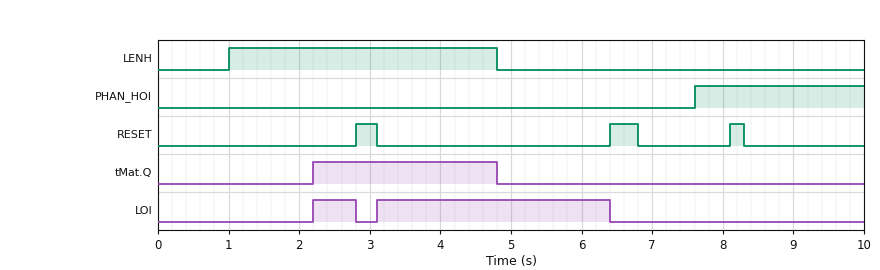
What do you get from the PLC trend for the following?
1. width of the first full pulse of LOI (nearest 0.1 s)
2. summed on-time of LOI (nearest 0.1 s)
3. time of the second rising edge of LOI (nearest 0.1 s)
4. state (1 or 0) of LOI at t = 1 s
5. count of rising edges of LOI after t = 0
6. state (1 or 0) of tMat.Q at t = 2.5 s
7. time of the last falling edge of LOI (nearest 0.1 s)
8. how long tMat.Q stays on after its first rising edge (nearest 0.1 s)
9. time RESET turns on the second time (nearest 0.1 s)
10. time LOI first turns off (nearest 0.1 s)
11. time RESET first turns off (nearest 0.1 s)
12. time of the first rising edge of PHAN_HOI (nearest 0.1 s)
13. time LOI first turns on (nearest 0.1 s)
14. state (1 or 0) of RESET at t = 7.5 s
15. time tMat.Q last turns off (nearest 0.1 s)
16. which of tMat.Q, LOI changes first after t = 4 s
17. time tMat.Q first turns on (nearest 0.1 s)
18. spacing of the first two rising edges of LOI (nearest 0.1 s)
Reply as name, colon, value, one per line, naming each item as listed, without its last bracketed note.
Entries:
width of the first full pulse of LOI: 0.6 s
summed on-time of LOI: 3.9 s
time of the second rising edge of LOI: 3.1 s
state (1 or 0) of LOI at t = 1 s: 0
count of rising edges of LOI after t = 0: 2
state (1 or 0) of tMat.Q at t = 2.5 s: 1
time of the last falling edge of LOI: 6.4 s
how long tMat.Q stays on after its first rising edge: 2.6 s
time RESET turns on the second time: 6.4 s
time LOI first turns off: 2.8 s
time RESET first turns off: 3.1 s
time of the first rising edge of PHAN_HOI: 7.6 s
time LOI first turns on: 2.2 s
state (1 or 0) of RESET at t = 7.5 s: 0
time tMat.Q last turns off: 4.8 s
which of tMat.Q, LOI changes first after t = 4 s: tMat.Q
time tMat.Q first turns on: 2.2 s
spacing of the first two rising edges of LOI: 0.9 s
